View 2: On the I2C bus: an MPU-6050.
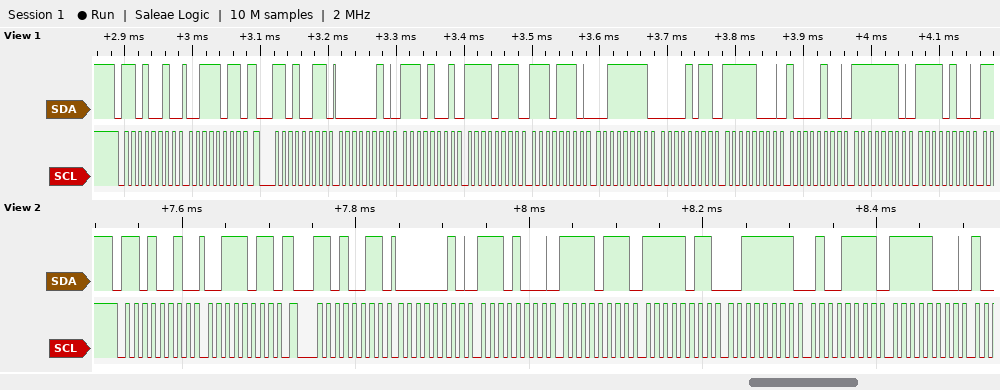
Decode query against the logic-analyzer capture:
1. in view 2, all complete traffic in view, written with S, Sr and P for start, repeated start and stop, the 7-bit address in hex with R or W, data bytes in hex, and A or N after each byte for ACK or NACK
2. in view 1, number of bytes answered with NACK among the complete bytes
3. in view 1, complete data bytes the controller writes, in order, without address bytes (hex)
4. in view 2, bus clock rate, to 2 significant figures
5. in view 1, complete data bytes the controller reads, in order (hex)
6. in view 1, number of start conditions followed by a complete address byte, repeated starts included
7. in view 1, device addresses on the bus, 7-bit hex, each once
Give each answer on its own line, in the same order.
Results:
S 69W A 3B A Sr 69R A 02 A E8 A F7 A FB A 3F A 4F A F8 A
0
3B
100 kHz
02 E9 F7 EE 3F 0B F8 84 FE F4
2
0x69
